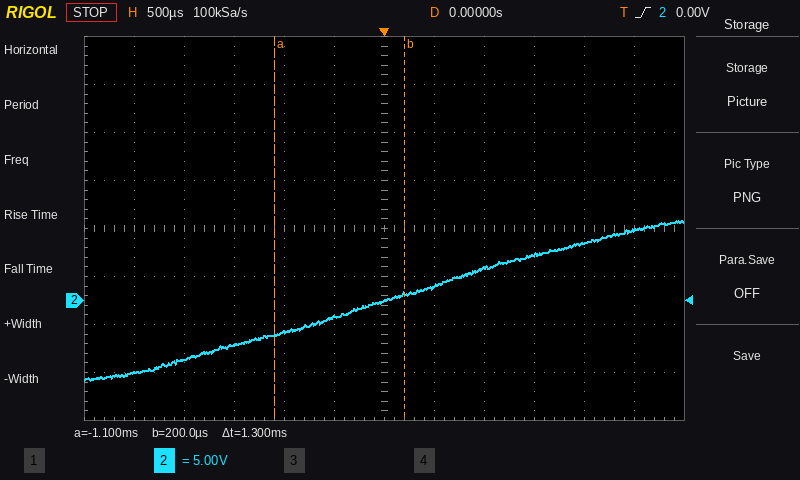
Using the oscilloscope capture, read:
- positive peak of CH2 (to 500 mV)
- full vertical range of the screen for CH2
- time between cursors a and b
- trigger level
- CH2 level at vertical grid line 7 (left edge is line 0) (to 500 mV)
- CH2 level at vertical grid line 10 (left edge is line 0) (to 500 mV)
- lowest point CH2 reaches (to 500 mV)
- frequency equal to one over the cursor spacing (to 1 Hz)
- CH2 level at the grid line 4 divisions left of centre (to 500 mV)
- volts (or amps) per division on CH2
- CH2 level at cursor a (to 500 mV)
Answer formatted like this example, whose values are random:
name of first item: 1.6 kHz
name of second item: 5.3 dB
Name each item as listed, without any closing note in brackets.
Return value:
positive peak of CH2: 8.5 V
full vertical range of the screen for CH2: 40 V
time between cursors a and b: 1.3 ms
trigger level: 0.00 V
CH2 level at vertical grid line 7 (left edge is line 0): 1.5 V
CH2 level at vertical grid line 10 (left edge is line 0): 6.0 V
lowest point CH2 reaches: -8.5 V
frequency equal to one over the cursor spacing: 769 Hz
CH2 level at the grid line 4 divisions left of centre: -6.0 V
volts (or amps) per division on CH2: 5 V
CH2 level at cursor a: -3.5 V
